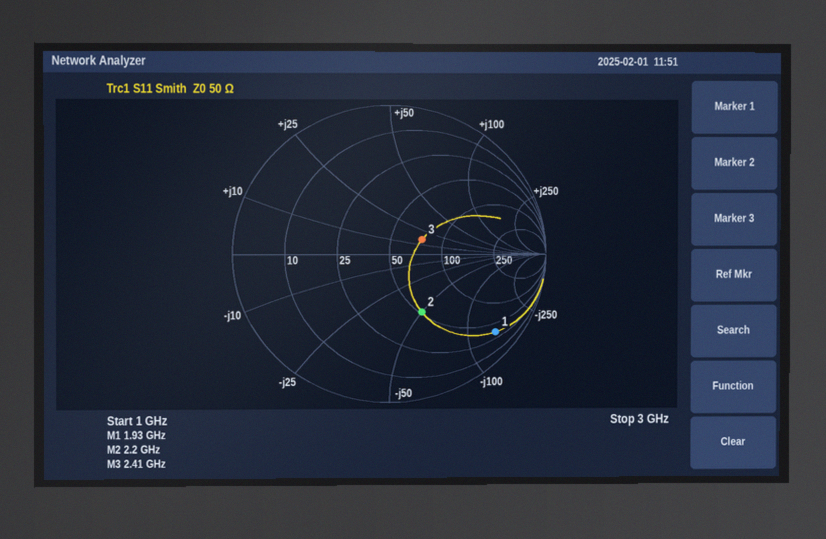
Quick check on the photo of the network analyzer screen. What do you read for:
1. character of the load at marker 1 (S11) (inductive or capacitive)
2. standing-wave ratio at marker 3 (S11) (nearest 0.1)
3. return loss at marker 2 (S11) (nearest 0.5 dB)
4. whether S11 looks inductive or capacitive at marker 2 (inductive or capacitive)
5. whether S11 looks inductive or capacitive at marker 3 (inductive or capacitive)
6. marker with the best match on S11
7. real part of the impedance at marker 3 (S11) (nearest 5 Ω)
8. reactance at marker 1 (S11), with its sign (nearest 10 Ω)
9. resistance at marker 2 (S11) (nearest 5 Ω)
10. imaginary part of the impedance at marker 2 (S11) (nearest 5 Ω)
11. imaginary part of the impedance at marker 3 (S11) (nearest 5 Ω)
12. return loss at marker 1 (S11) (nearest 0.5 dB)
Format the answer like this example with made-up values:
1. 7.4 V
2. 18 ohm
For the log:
1. capacitive
2. 1.6
3. 7.0 dB
4. capacitive
5. inductive
6. marker 3
7. 75 Ω
8. -140 Ω
9. 50 Ω
10. -50 Ω
11. +15 Ω
12. 1.5 dB
